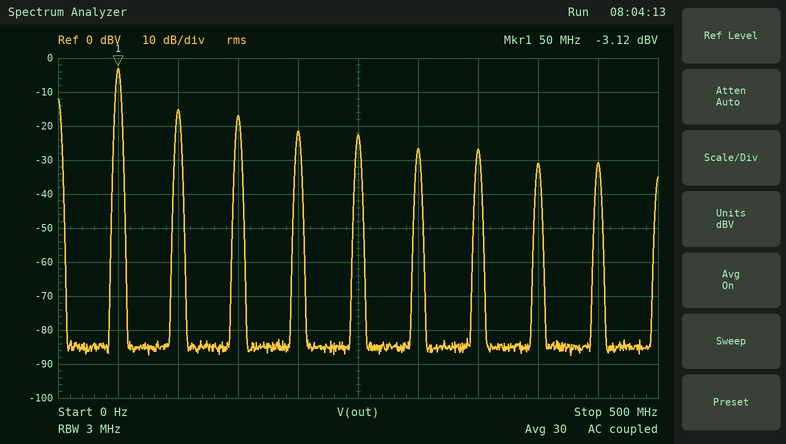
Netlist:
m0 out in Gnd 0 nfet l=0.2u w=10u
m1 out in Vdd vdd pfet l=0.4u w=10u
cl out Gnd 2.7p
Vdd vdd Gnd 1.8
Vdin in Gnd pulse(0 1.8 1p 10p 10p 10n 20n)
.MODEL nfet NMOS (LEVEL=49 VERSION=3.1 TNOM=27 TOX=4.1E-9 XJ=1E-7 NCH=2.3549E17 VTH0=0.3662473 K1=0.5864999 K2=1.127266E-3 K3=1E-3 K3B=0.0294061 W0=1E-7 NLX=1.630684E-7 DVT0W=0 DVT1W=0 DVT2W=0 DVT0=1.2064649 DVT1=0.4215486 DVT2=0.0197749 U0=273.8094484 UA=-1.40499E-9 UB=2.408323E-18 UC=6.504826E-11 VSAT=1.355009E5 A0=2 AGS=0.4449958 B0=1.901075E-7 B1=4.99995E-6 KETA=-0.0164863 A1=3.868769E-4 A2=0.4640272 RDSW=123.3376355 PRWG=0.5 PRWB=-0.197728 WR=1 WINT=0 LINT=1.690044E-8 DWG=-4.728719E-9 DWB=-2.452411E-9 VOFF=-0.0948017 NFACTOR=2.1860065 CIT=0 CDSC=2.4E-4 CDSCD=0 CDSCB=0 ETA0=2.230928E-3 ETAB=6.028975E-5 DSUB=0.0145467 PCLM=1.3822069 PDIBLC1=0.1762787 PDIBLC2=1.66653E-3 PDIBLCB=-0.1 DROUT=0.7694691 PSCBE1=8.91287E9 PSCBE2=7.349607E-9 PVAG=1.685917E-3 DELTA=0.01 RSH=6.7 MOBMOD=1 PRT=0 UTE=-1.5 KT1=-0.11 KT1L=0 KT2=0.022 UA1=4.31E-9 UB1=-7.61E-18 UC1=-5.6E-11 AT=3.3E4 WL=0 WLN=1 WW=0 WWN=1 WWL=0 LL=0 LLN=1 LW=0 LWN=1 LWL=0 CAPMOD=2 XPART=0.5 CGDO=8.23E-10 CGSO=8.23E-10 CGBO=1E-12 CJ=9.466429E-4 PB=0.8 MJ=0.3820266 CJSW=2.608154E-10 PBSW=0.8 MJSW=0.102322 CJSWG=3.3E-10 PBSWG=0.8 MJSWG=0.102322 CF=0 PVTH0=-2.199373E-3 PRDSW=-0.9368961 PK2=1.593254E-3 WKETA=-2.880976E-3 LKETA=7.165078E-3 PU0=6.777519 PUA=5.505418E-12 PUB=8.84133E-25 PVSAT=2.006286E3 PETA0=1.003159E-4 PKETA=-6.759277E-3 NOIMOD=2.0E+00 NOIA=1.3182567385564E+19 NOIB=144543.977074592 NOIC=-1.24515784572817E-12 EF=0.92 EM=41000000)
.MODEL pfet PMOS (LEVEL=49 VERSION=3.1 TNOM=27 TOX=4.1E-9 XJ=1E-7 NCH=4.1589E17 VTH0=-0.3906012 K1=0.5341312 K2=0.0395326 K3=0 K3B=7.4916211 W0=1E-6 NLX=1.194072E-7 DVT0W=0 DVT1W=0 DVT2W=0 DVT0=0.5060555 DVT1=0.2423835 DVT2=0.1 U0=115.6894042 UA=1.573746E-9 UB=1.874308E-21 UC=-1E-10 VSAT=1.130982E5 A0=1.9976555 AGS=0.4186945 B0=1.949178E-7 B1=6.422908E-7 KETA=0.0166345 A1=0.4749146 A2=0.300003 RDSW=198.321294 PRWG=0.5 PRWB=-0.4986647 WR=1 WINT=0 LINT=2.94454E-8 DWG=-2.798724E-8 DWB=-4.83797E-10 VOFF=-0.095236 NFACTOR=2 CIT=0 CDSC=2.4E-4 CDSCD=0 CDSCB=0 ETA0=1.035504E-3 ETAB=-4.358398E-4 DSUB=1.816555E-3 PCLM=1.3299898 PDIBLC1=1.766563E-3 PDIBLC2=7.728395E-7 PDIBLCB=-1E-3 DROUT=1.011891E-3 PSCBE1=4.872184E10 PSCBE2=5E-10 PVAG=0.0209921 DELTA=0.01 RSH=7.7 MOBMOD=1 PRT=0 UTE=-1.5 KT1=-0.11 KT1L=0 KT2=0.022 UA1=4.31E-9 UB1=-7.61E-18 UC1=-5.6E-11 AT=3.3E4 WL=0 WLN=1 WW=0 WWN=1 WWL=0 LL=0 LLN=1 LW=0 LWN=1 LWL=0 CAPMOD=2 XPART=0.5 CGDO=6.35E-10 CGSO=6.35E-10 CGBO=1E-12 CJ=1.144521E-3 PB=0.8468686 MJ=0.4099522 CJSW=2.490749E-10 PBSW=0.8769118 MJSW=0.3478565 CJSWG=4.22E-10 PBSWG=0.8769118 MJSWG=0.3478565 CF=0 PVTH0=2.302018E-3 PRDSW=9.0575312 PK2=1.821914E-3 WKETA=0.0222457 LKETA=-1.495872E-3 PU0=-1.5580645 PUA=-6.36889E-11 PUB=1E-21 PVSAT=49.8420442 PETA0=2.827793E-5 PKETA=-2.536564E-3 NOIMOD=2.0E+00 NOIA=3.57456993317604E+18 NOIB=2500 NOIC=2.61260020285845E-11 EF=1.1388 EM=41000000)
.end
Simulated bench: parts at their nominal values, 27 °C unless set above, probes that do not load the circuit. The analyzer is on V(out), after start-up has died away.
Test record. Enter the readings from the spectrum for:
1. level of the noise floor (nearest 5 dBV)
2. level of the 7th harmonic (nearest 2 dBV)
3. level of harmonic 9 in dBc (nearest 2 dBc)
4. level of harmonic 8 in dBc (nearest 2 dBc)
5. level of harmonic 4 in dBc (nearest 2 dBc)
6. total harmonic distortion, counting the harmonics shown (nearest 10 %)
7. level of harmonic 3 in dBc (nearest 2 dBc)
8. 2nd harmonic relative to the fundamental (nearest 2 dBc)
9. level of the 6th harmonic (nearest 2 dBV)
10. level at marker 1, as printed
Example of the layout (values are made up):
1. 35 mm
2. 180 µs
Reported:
1. -85 dBV
2. -26 dBV
3. -28 dBc
4. -28 dBc
5. -18 dBc
6. 40 %
7. -14 dBc
8. -12 dBc
9. -26 dBV
10. -3.12 dBV
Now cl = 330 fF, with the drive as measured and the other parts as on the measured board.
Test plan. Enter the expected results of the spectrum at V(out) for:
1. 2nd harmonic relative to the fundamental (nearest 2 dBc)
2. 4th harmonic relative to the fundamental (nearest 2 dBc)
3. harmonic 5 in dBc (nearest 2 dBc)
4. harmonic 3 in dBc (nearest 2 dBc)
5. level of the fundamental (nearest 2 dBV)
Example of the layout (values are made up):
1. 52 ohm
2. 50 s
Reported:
1. -26 dBc
2. -26 dBc
3. -14 dBc
4. -10 dBc
5. -2 dBV
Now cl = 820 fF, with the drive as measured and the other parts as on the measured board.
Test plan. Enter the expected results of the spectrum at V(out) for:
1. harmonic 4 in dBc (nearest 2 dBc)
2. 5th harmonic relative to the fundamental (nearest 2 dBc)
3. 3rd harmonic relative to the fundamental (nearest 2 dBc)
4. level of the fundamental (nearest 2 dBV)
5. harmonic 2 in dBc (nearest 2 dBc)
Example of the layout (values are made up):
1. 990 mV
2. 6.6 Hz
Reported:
1. -20 dBc
2. -16 dBc
3. -10 dBc
4. -2 dBV
5. -20 dBc
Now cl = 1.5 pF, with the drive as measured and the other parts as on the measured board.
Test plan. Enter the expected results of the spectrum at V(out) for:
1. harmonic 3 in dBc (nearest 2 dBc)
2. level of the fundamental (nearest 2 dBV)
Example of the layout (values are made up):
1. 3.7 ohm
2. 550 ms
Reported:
1. -12 dBc
2. -2 dBV
